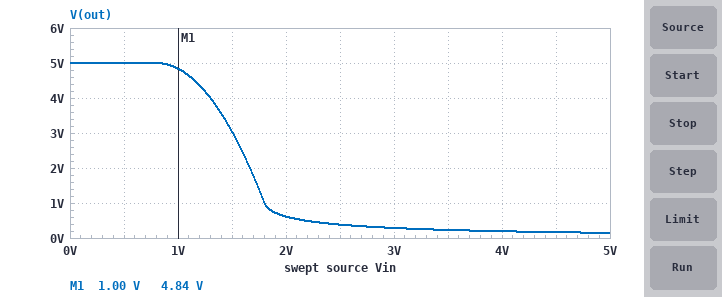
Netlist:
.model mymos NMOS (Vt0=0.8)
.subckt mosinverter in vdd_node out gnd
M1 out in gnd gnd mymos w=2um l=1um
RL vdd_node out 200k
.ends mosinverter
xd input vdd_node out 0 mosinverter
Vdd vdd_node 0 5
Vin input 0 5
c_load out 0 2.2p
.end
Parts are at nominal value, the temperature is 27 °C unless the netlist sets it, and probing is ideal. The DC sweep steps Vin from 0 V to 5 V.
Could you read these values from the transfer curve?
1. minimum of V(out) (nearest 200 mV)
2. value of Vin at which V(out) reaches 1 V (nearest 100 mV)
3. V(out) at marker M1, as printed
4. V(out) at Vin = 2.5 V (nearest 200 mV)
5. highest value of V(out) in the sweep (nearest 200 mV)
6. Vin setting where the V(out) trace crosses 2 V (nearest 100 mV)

200 mV
1.8 V
4.84 V
400 mV
5.0 V
1.7 V
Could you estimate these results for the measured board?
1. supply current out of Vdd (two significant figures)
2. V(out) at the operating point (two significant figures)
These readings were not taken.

24 µA
150 mV
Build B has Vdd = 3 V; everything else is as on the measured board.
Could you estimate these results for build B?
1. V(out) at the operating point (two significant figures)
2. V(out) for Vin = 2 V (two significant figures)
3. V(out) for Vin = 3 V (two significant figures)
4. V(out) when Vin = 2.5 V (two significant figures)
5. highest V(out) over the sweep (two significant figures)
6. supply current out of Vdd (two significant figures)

88 mV
320 mV
170 mV
220 mV
3.0 V
15 µA
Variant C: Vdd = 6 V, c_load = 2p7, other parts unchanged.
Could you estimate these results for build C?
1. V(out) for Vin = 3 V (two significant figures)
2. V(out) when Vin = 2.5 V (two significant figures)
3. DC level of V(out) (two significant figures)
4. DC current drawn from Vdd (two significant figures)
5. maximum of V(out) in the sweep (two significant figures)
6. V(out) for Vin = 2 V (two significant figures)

350 mV
470 mV
180 mV
29 µA
6.0 V
820 mV
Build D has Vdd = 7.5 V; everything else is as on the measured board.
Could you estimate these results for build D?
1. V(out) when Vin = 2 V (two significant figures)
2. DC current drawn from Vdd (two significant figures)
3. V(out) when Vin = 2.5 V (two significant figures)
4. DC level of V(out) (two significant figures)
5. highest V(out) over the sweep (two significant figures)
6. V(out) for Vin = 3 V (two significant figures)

1.7 V
36 µA
620 mV
220 mV
7.5 V
450 mV
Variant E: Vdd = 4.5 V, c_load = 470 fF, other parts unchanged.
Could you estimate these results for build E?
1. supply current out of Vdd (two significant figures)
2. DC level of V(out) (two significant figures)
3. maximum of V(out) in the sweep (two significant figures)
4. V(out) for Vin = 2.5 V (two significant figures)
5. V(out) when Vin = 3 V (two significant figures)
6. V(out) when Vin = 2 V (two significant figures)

22 µA
130 mV
4.5 V
340 mV
260 mV
530 mV
